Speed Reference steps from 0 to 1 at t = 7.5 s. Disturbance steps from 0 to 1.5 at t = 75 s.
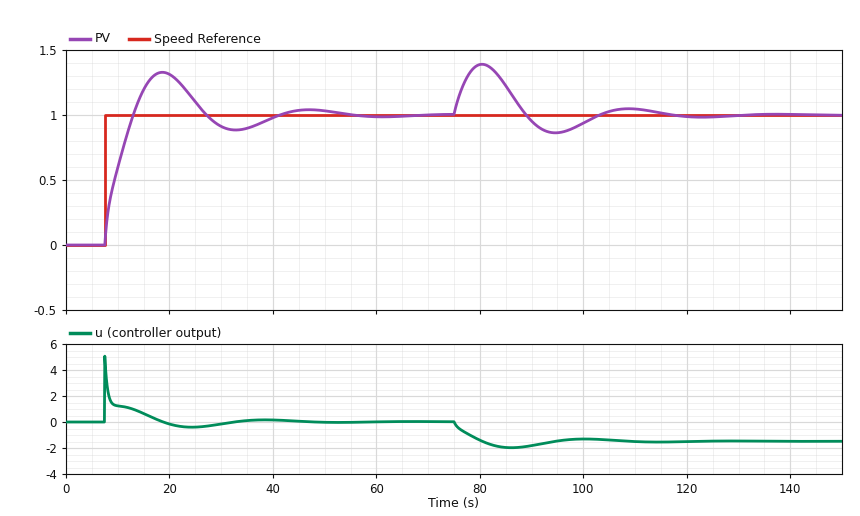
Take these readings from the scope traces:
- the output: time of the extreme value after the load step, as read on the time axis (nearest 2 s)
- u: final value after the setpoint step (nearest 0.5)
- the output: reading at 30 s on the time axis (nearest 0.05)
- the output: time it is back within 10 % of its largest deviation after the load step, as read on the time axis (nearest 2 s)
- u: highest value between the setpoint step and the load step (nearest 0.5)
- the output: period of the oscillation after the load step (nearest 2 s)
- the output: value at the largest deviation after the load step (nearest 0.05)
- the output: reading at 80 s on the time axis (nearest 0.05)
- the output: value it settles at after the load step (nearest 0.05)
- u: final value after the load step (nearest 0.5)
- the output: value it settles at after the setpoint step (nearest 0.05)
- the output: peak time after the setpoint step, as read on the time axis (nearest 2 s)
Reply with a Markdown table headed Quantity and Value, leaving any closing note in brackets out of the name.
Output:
| Quantity | Value |
|---|---|
| the output: time of the extreme value after the load step, as read on the time axis | 80 s |
| u: final value after the setpoint step | 0.0 |
| the output: reading at 30 s on the time axis | 0.90 |
| the output: time it is back within 10 % of its largest deviation after the load step, as read on the time axis | 112 s |
| u: highest value between the setpoint step and the load step | 5.0 |
| the output: period of the oscillation after the load step | 28 s |
| the output: value at the largest deviation after the load step | 1.40 |
| the output: reading at 80 s on the time axis | 1.40 |
| the output: value it settles at after the load step | 1.00 |
| u: final value after the load step | -1.5 |
| the output: value it settles at after the setpoint step | 1.00 |
| the output: peak time after the setpoint step, as read on the time axis | 18 s |
